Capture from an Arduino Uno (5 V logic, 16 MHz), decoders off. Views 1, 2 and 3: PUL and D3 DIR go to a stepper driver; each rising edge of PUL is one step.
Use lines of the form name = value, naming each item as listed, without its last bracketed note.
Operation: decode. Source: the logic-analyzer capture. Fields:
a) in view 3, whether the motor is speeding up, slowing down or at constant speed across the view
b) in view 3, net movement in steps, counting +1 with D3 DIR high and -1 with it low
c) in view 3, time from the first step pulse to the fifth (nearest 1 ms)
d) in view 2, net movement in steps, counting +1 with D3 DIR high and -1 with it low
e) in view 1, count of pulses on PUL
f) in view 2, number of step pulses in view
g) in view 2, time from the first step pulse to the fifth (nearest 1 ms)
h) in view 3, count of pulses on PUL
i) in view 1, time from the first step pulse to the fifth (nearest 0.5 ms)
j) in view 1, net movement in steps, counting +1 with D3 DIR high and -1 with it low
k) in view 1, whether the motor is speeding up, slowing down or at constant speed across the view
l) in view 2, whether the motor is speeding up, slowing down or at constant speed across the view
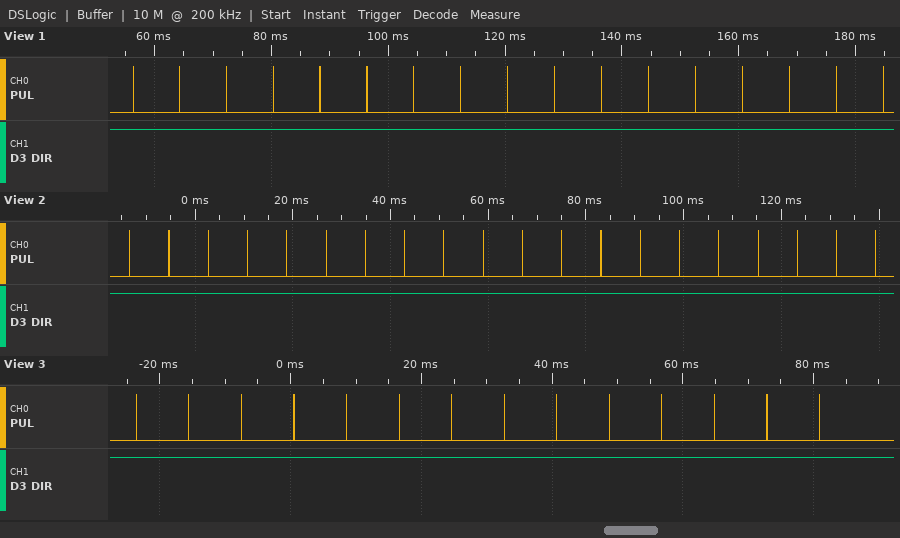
in view 3, whether the motor is speeding up, slowing down or at constant speed across the view = constant speed
in view 3, net movement in steps, counting +1 with D3 DIR high and -1 with it low = +14
in view 3, time from the first step pulse to the fifth = 32 ms
in view 2, net movement in steps, counting +1 with D3 DIR high and -1 with it low = +20
in view 1, count of pulses on PUL = 17
in view 2, number of step pulses in view = 20
in view 2, time from the first step pulse to the fifth = 32 ms
in view 3, count of pulses on PUL = 14
in view 1, time from the first step pulse to the fifth = 32.0 ms
in view 1, net movement in steps, counting +1 with D3 DIR high and -1 with it low = +17
in view 1, whether the motor is speeding up, slowing down or at constant speed across the view = constant speed
in view 2, whether the motor is speeding up, slowing down or at constant speed across the view = constant speed
